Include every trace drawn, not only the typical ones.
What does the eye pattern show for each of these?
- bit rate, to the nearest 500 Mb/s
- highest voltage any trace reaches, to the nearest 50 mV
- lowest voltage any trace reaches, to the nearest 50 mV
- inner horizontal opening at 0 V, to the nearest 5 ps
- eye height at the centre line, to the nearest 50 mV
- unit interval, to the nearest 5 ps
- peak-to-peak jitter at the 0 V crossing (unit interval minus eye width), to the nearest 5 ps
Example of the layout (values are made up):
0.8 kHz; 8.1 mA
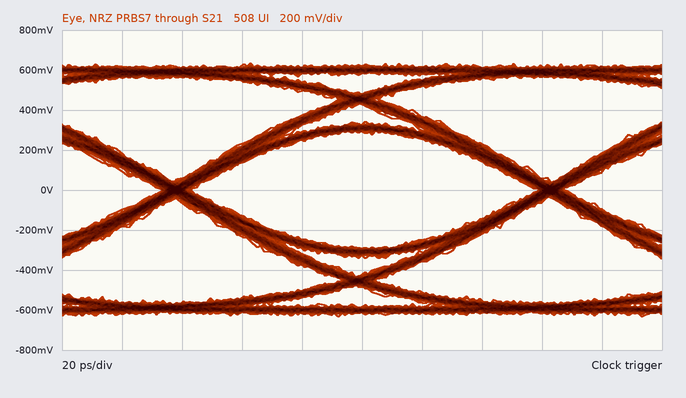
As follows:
8.0 Gb/s; 650 mV; -650 mV; 115 ps; 600 mV; 125 ps; 10 ps
